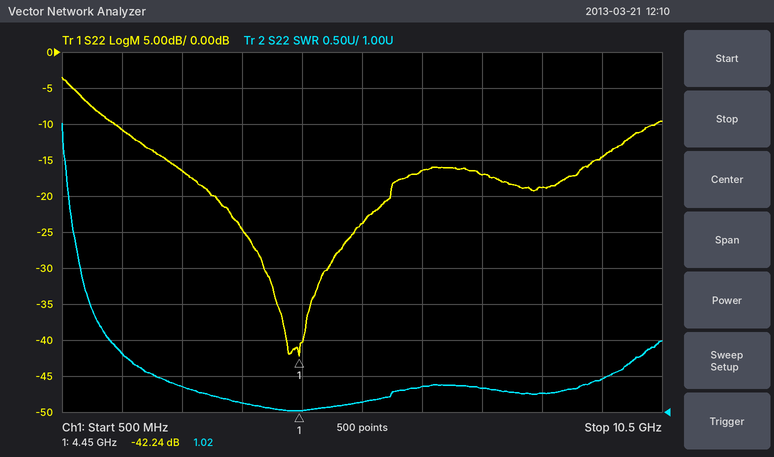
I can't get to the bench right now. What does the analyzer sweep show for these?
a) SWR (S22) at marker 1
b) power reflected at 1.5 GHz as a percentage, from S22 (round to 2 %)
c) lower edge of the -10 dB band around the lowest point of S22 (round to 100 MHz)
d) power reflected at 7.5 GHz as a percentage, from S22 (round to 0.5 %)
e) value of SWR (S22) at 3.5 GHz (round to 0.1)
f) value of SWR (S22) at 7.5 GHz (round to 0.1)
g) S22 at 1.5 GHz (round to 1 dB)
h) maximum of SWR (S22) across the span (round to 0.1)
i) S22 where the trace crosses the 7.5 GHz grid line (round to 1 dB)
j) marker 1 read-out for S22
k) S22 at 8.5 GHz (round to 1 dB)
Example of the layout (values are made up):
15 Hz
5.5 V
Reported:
1.02
8 %
1.4 GHz
2.0 %
1.1
1.3
-11 dB
5.0
-17 dB
-42.24 dB
-19 dB
